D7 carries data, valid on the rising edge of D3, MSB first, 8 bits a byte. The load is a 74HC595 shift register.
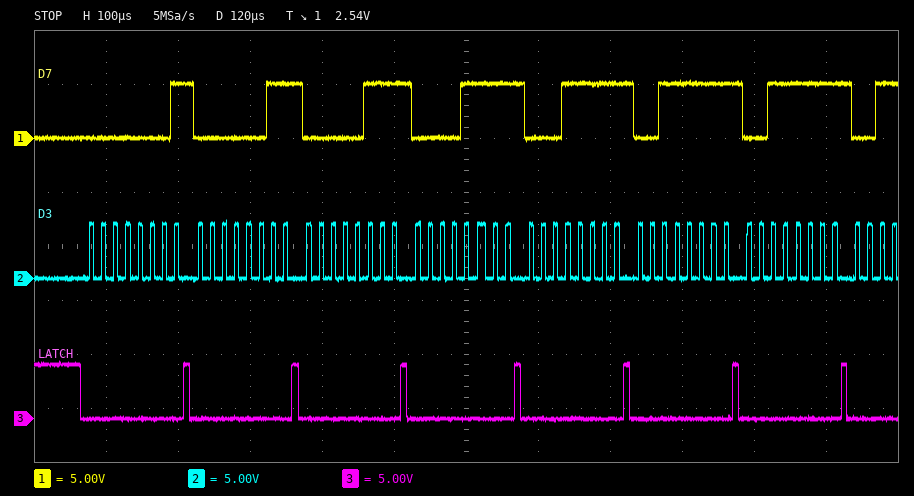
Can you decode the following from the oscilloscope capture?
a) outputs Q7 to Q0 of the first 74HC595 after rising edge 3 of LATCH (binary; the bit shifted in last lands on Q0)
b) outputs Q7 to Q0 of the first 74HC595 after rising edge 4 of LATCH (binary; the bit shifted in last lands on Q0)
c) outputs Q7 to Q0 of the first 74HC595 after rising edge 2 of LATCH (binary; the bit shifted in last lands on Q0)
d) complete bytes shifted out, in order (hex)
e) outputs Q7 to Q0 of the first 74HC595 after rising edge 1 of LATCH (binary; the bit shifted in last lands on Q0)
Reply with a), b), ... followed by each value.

a) 00000111
b) 00001111
c) 00000011
d) 01 03 07 0F 1F 3F 3F
e) 00000001
